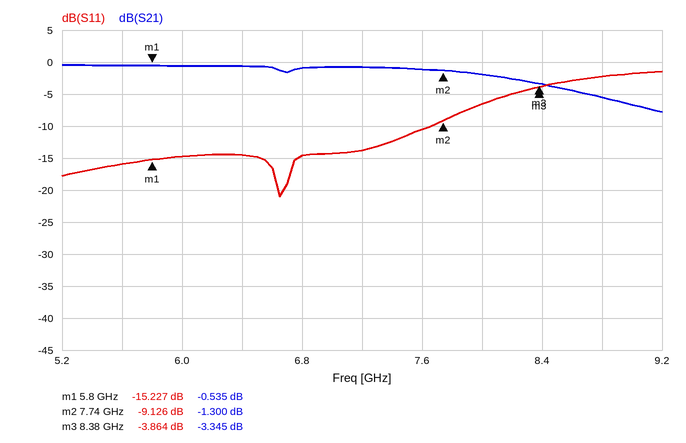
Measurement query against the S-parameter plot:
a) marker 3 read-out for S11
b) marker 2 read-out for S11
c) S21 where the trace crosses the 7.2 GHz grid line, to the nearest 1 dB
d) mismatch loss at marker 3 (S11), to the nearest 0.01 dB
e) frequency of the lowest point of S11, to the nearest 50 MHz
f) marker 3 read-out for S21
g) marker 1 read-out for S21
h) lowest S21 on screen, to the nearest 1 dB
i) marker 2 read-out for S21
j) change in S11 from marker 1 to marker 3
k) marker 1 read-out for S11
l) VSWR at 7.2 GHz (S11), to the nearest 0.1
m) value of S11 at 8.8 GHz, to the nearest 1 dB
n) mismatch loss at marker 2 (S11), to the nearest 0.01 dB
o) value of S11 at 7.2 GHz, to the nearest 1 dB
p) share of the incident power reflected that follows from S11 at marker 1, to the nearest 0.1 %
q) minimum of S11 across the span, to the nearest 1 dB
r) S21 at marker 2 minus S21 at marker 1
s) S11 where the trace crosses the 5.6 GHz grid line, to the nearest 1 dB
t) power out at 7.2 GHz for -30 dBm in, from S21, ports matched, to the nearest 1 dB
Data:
-3.864 dB
-9.126 dB
-1 dB
2.30 dB
6.65 GHz
-3.345 dB
-0.535 dB
-8 dB
-1.300 dB
11.363 dB
-15.227 dB
1.5
-2 dB
0.57 dB
-14 dB
3.0 %
-21 dB
-0.765 dB
-16 dB
-31 dBm
